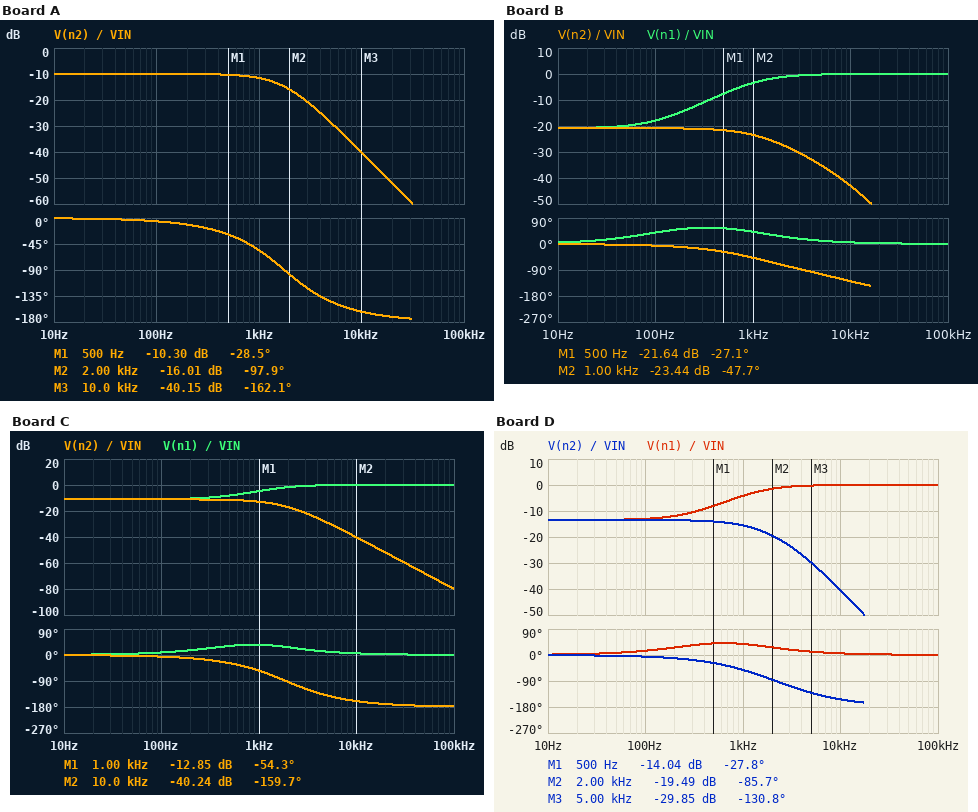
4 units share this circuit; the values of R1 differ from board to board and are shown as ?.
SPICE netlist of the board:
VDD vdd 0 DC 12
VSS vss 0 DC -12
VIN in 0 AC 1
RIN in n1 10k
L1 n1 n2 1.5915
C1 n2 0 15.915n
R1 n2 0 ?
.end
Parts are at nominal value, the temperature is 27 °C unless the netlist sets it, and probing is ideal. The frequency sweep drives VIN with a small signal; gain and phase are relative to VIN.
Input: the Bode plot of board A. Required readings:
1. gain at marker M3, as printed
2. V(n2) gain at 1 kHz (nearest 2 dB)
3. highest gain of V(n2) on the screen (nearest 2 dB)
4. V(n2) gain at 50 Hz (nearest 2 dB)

-40.15 dB
-12 dB
-10 dB
-10 dB
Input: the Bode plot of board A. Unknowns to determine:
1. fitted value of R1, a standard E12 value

4.7 kΩ
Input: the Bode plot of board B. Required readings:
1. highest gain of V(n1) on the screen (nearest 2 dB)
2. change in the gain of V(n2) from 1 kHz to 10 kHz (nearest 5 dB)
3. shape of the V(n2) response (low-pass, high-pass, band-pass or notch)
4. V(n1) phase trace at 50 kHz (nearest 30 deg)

0 dB
-20 dB
low-pass
0 deg
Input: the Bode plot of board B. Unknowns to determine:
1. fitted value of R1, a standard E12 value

1 kΩ
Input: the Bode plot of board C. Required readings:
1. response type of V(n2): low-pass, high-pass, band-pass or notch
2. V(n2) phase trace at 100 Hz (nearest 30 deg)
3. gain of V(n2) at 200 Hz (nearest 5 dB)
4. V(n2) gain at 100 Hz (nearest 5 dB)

low-pass
0 deg
-10 dB
-10 dB
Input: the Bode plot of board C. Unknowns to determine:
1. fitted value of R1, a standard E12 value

3.9 kΩ
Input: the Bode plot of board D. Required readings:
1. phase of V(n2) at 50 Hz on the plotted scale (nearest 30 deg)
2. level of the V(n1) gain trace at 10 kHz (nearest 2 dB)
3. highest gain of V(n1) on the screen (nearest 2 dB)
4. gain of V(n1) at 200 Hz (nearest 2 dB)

0 deg
0 dB
0 dB
-12 dB
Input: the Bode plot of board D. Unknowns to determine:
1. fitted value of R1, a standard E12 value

2.7 kΩ
